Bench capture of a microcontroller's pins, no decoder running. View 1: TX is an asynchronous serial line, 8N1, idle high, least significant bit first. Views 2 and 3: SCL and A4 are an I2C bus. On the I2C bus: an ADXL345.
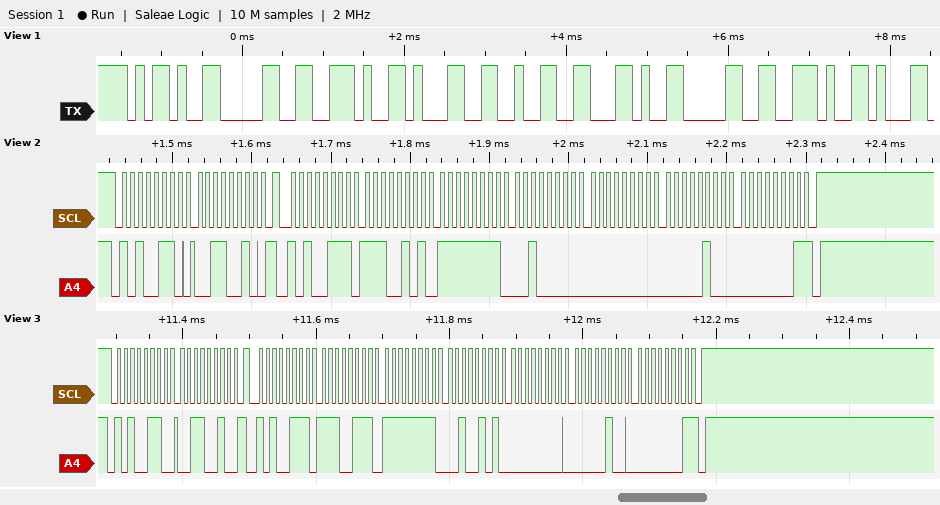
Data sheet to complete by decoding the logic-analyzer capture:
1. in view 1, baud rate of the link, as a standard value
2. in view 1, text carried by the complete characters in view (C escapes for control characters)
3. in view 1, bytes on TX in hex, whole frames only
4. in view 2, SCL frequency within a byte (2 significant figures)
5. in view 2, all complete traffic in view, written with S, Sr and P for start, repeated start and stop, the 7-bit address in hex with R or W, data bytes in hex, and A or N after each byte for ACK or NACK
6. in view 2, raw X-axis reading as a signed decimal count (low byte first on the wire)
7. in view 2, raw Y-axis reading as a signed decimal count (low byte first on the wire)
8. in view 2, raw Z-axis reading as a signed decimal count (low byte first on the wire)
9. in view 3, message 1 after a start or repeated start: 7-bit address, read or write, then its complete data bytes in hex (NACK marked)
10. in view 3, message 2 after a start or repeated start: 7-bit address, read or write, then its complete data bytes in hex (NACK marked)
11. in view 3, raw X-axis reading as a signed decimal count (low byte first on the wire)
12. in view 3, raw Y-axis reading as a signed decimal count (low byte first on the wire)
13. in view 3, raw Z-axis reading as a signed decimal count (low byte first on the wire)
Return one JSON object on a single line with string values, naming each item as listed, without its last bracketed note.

{"in view 1, baud rate of the link, as a standard value": "9600 baud", "in view 1, text carried by the complete characters in view": "\"-0.12,0.\"", "in view 1, bytes on TX in hex, whole frames only": "2D 30 2E 31 32 2C 30 2E", "in view 2, SCL frequency within a byte": "100 kHz", "in view 2, all complete traffic in view, written with S, Sr and P for start, repeated start and stop, the 7-bit address in hex with R or W, data bytes in hex, and A or N after each byte for ACK or NACK": "S 53W A 32 A Sr 53R A E5 A FF A 20 A 00 A 04 A 01 N P", "in view 2, raw X-axis reading as a signed decimal count": "-27", "in view 2, raw Y-axis reading as a signed decimal count": "32", "in view 2, raw Z-axis reading as a signed decimal count": "260", "in view 3, message 1 after a start or repeated start: 7-bit address, read or write, then its complete data bytes in hex": "0x53 write: 32", "in view 3, message 2 after a start or repeated start: 7-bit address, read or write, then its complete data bytes in hex": "0x53 read: E7 FF 25 00 04 01 NACK", "in view 3, raw X-axis reading as a signed decimal count": "-25", "in view 3, raw Y-axis reading as a signed decimal count": "37", "in view 3, raw Z-axis reading as a signed decimal count": "260"}
